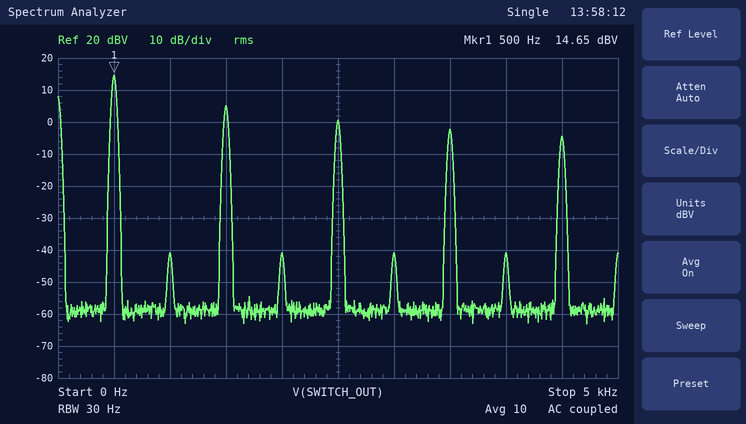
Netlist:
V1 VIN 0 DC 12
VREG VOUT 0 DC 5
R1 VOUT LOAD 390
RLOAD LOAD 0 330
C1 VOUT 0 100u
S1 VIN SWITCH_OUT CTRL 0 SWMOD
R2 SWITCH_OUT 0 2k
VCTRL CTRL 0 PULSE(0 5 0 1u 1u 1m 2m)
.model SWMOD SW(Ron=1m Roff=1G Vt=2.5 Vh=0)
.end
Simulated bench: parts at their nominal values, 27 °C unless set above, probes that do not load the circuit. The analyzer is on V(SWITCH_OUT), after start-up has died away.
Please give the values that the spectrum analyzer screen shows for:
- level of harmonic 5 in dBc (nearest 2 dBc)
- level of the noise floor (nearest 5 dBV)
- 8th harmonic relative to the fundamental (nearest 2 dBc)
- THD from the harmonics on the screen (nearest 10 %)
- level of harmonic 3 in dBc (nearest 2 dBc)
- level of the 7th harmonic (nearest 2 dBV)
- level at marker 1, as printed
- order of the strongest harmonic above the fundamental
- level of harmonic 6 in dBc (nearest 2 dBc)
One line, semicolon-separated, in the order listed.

-14 dBc; -60 dBV; -56 dBc; 40 %; -10 dBc; -2 dBV; 14.65 dBV; 3; -56 dBc
